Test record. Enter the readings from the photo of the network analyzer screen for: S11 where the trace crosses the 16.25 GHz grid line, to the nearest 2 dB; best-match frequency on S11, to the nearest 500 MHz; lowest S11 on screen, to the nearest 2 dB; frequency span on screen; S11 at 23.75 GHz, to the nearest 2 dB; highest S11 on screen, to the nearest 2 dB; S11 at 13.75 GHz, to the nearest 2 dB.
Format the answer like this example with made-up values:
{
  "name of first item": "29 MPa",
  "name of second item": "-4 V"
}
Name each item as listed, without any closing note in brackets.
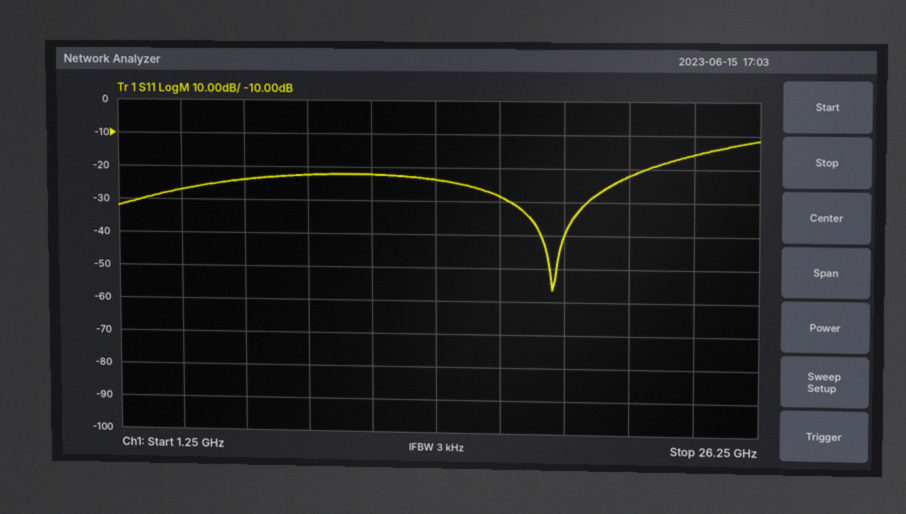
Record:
{
  "S11 where the trace crosses the 16.25 GHz grid line, to the nearest 2 dB": "-28 dB",
  "best-match frequency on S11, to the nearest 500 MHz": "18.5 GHz",
  "lowest S11 on screen, to the nearest 2 dB": "-56 dB",
  "frequency span on screen": "25 GHz",
  "S11 at 23.75 GHz, to the nearest 2 dB": "-16 dB",
  "highest S11 on screen, to the nearest 2 dB": "-12 dB",
  "S11 at 13.75 GHz, to the nearest 2 dB": "-24 dB"
}
